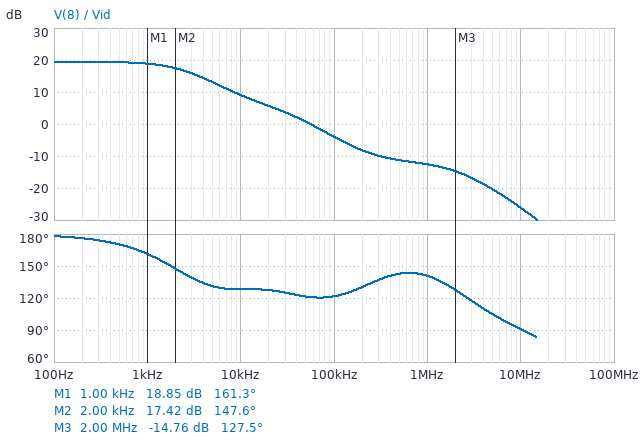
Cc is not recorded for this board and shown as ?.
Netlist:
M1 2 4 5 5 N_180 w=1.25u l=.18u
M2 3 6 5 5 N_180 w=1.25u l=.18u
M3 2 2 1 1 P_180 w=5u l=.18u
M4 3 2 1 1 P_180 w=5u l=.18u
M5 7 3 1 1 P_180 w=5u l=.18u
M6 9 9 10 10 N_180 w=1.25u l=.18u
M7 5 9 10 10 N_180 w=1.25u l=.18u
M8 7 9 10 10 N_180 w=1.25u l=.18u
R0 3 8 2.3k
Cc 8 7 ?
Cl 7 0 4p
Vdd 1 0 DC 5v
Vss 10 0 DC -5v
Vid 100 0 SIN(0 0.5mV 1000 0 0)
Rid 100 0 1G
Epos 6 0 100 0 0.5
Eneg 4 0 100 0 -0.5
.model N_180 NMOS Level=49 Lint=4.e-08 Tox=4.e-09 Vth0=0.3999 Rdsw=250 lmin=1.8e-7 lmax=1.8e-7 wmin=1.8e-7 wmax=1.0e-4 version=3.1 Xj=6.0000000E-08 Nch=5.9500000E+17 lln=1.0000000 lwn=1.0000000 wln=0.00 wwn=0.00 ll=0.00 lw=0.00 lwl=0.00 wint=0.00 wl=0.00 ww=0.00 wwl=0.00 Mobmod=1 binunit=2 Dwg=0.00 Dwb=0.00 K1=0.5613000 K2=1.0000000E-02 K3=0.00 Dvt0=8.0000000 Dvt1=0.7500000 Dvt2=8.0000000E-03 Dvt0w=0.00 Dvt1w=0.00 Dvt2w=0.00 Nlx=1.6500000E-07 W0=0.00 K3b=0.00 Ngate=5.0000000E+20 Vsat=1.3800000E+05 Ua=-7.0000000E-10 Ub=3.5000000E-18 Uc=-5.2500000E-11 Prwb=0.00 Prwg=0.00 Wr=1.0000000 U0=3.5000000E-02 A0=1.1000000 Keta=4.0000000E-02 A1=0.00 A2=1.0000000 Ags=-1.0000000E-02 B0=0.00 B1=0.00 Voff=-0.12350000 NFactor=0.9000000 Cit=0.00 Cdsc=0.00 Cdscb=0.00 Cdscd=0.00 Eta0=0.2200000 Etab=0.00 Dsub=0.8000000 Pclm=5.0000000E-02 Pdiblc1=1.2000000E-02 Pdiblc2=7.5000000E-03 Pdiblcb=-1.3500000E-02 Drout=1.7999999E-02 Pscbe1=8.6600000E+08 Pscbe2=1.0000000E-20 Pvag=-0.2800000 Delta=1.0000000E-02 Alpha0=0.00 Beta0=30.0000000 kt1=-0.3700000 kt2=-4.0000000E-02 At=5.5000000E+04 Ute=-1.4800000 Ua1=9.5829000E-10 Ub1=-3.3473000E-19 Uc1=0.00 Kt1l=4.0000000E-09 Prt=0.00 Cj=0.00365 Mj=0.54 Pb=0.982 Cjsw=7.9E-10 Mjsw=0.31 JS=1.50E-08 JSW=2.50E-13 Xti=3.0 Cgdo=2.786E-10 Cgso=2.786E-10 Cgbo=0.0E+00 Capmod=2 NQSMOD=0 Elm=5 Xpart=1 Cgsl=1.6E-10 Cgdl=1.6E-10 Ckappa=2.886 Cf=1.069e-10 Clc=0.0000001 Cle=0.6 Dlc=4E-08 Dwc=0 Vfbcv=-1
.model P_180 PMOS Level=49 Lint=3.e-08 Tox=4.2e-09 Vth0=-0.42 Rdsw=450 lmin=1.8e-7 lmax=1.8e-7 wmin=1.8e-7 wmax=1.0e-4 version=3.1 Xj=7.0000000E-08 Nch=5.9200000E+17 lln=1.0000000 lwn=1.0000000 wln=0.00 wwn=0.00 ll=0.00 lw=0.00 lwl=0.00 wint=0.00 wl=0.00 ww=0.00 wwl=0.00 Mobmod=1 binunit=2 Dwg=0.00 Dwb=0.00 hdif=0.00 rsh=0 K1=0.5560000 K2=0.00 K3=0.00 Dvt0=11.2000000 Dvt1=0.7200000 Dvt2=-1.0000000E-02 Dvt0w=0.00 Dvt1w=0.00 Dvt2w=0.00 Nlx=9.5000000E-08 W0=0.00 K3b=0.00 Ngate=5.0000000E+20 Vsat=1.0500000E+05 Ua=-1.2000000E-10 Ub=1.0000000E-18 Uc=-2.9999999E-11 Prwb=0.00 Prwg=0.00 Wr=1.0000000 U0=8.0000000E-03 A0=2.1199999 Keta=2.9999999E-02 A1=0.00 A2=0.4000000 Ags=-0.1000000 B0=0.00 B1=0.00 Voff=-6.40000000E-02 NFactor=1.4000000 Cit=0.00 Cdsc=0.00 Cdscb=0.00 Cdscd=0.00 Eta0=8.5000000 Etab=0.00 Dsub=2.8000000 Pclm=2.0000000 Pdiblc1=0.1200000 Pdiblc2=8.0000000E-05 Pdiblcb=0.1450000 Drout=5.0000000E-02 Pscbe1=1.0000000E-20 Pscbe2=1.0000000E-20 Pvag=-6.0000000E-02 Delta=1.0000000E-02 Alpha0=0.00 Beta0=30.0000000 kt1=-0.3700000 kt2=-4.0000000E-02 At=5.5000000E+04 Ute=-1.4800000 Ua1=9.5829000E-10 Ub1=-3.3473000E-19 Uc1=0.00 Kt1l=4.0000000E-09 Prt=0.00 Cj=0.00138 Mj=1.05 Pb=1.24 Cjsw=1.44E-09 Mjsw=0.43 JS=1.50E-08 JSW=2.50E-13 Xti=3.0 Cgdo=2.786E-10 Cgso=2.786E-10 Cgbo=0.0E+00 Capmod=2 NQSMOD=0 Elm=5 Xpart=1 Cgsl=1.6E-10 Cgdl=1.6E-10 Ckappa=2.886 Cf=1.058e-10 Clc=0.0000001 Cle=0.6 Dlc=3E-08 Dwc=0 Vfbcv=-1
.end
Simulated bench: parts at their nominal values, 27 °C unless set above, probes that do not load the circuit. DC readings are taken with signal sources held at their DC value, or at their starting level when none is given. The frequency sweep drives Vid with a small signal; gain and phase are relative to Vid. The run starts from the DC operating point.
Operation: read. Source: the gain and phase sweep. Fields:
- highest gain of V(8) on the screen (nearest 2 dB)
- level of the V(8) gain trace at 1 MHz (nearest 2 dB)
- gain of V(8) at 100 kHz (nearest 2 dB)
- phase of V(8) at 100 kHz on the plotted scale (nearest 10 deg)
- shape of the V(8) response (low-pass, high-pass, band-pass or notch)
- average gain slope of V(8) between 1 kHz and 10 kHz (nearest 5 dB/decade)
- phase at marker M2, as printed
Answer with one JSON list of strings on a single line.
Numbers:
["20 dB", "-12 dB", "-4 dB", "120 deg", "low-pass", "-10 dB/decade", "147.6 deg"]
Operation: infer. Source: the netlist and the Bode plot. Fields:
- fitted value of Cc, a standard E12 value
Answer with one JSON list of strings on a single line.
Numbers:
["2.2 pF"]
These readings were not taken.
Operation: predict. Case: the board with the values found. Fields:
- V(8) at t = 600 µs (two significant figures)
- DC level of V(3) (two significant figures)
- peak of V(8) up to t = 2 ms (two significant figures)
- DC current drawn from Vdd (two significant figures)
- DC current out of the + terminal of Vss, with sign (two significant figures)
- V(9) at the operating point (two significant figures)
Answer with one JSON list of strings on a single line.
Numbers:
["4.8 V", "4.8 V", "4.8 V", "2.1 µA", "-2.1 µA", "-5.0 V"]
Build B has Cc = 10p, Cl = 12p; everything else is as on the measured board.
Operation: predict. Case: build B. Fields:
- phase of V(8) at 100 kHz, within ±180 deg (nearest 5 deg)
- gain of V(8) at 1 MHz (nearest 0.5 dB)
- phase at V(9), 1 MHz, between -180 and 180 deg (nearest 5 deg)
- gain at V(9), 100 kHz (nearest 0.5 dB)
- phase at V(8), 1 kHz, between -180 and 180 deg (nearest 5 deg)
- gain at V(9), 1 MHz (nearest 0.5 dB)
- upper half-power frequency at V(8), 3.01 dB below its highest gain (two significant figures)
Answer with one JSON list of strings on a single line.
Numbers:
["145 deg", "-19.0 dB", "155 deg", "-23.0 dB", "125 deg", "-44.5 dB", "550 Hz"]
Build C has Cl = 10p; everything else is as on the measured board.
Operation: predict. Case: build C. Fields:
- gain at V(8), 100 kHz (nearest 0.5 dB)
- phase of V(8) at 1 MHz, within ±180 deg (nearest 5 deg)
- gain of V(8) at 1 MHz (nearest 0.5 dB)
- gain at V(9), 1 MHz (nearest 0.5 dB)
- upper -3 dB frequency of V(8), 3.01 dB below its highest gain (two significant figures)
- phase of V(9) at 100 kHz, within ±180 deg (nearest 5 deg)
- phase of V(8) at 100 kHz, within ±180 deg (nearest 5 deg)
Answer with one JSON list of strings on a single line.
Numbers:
["-2.0 dB", "125 deg", "-10.0 dB", "-33.5 dB", "2.5 kHz", "-80 deg", "135 deg"]
